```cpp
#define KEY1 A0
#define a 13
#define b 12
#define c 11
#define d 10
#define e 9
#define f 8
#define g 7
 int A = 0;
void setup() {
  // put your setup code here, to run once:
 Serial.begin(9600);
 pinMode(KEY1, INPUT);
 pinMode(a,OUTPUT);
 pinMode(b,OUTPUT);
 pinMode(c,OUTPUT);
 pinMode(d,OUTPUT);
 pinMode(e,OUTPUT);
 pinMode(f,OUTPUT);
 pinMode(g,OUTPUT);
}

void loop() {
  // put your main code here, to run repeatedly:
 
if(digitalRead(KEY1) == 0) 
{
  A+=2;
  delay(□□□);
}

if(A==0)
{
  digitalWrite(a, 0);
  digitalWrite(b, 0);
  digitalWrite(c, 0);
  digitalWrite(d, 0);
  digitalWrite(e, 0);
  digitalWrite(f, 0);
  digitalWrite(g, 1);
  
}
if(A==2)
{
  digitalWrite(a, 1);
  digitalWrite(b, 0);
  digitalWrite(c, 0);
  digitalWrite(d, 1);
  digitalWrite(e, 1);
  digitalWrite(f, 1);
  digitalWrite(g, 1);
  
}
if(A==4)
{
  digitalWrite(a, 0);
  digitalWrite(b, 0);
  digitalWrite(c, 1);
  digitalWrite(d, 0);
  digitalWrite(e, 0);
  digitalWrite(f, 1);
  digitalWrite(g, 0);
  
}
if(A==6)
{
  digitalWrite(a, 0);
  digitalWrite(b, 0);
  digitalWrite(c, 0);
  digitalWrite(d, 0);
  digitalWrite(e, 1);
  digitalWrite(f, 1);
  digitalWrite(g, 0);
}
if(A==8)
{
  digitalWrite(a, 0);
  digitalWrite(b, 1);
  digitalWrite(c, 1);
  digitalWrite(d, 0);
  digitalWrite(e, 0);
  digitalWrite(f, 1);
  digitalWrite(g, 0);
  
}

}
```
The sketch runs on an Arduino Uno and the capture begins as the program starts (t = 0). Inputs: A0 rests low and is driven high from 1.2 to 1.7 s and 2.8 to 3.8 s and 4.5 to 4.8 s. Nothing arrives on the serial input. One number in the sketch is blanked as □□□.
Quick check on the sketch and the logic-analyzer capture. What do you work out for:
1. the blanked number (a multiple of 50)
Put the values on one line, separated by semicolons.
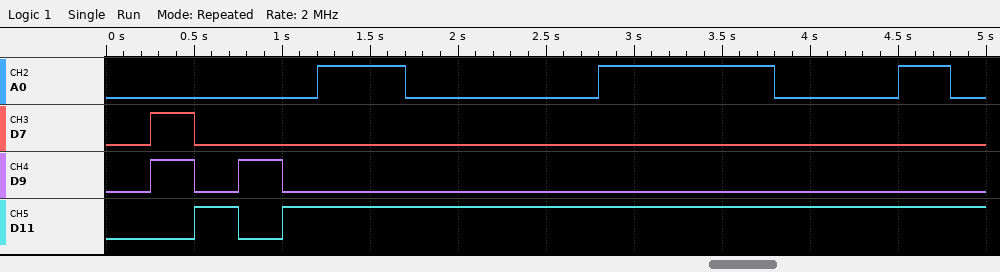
250
